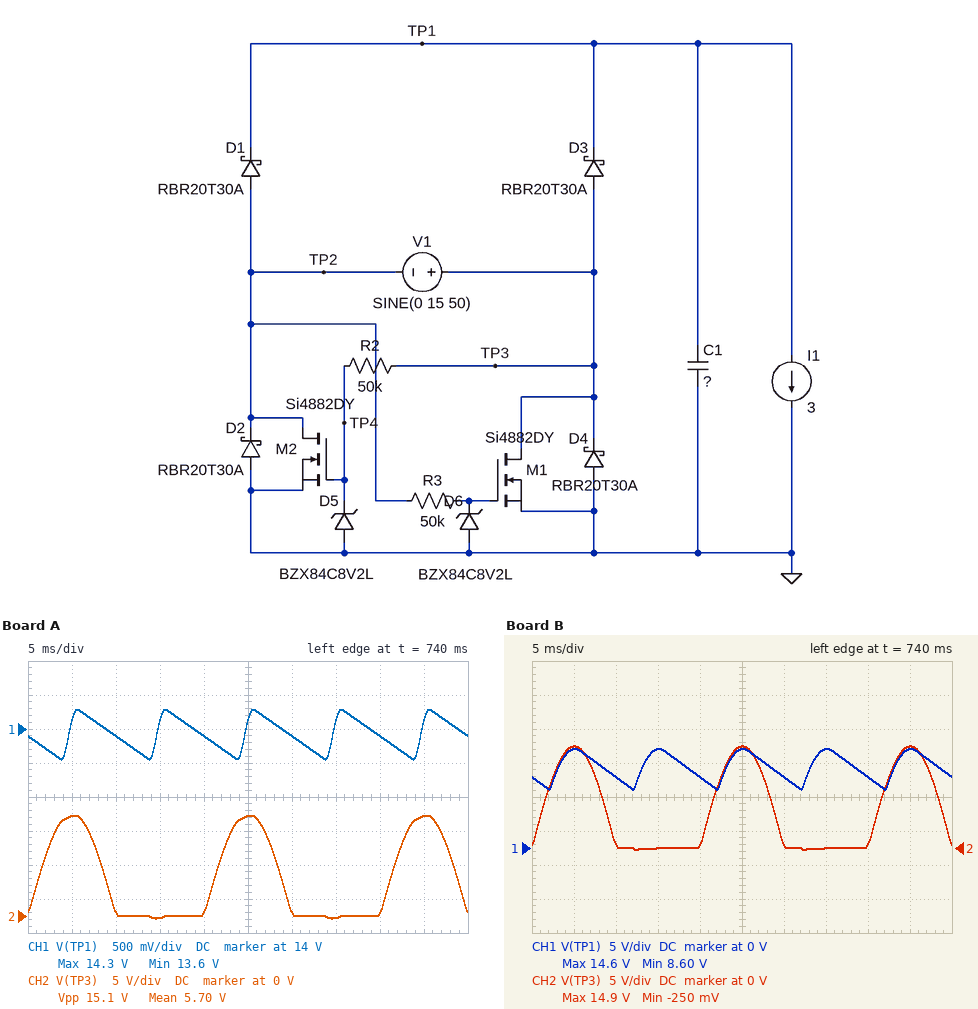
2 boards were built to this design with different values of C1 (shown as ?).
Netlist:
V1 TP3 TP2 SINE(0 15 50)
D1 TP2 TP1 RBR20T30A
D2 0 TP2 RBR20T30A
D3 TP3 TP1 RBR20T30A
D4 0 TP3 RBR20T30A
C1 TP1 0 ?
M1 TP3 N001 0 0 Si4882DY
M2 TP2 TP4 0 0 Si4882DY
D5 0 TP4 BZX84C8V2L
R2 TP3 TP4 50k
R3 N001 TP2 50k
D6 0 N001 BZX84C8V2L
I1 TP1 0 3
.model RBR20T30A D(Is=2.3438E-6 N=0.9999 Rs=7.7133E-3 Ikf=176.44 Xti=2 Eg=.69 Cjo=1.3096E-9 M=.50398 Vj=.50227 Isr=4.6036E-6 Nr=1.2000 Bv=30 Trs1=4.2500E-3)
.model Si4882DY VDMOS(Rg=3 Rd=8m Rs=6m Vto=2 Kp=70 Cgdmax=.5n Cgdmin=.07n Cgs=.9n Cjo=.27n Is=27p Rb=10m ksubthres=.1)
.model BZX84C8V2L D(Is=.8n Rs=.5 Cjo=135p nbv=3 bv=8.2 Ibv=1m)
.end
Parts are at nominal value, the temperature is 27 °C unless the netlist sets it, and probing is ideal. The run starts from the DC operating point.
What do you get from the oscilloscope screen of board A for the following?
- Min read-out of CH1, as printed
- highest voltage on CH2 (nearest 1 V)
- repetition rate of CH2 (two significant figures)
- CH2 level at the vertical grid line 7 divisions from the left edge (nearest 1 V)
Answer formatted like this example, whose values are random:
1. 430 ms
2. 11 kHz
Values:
1. 13.6 V
2. 15 V
3. 50 Hz
4. 0 V
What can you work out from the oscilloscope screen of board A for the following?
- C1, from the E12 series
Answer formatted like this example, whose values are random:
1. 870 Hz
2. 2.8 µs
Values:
1. 33 mF
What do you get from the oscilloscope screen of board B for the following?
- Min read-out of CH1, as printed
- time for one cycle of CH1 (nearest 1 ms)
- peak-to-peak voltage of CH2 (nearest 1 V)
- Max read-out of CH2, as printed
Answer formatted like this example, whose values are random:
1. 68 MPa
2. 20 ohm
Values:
1. 8.60 V
2. 10 ms
3. 15 V
4. 14.9 V
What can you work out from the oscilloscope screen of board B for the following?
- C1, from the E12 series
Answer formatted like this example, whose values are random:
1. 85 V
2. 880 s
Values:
1. 3.3 mF
